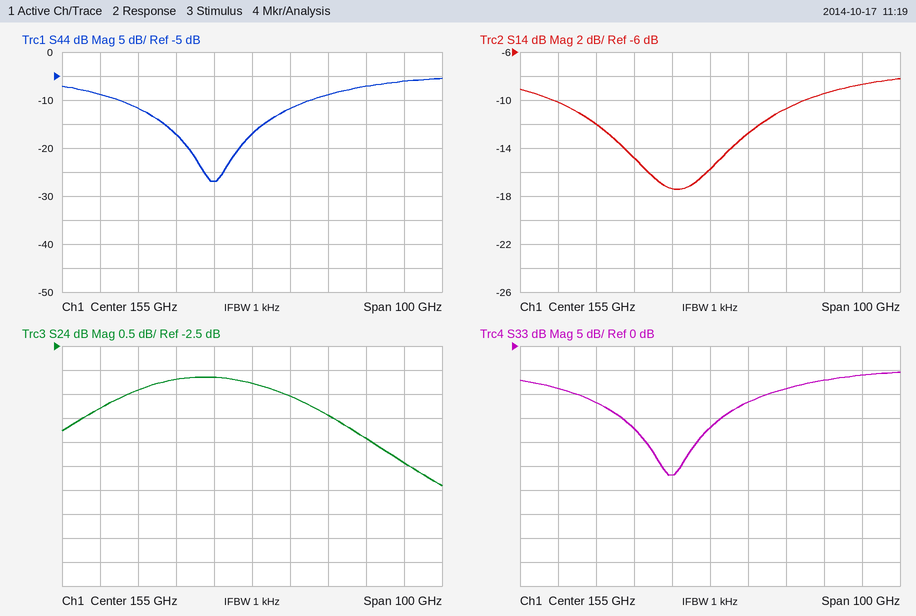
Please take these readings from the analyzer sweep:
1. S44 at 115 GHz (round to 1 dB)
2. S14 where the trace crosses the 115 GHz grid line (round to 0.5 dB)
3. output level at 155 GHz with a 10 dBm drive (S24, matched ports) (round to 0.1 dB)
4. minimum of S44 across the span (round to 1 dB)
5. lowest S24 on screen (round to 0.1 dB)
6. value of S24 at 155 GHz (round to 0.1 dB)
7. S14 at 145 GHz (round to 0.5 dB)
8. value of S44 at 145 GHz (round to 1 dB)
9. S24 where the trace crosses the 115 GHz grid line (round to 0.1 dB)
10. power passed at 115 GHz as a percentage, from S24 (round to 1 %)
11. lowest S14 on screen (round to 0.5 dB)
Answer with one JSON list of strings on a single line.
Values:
["-9 dB", "-10.0 dB", "6.7 dBm", "-27 dB", "-5.4 dB", "-3.3 dB", "-17.5 dB", "-27 dB", "-3.8 dB", "42 %", "-17.5 dB"]
